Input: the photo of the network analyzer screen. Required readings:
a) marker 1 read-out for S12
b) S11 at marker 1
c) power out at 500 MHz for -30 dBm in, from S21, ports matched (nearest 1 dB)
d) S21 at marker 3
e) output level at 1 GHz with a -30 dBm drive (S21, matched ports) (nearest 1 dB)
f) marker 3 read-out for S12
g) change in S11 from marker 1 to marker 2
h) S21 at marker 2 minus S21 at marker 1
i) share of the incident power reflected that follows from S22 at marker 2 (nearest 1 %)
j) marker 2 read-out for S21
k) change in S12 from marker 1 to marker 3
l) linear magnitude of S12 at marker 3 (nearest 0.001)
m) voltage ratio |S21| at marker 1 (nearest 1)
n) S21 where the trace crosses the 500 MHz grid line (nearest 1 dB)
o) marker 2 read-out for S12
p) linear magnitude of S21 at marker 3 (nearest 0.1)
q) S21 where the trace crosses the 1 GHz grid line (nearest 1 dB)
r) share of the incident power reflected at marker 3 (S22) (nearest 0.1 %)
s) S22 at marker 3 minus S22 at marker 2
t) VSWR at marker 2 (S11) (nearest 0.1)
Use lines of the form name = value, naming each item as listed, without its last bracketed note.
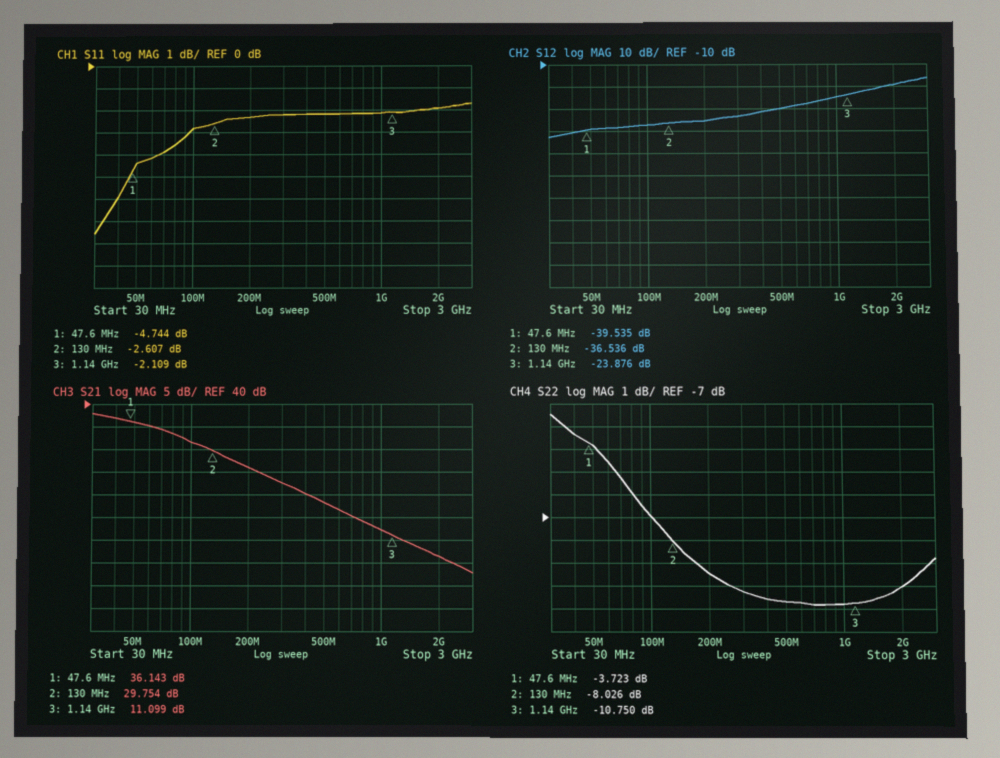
marker 1 read-out for S12 = -39.535 dB
S11 at marker 1 = -4.744 dB
power out at 500 MHz for -30 dBm in, from S21, ports matched = -12 dBm
S21 at marker 3 = 11.099 dB
output level at 1 GHz with a -30 dBm drive (S21, matched ports) = -18 dBm
marker 3 read-out for S12 = -23.876 dB
change in S11 from marker 1 to marker 2 = 2.137 dB
S21 at marker 2 minus S21 at marker 1 = -6.389 dB
share of the incident power reflected that follows from S22 at marker 2 = 16 %
marker 2 read-out for S21 = 29.754 dB
change in S12 from marker 1 to marker 3 = 15.659 dB
linear magnitude of S12 at marker 3 = 0.064
voltage ratio |S21| at marker 1 = 64
S21 where the trace crosses the 500 MHz grid line = 18 dB
marker 2 read-out for S12 = -36.536 dB
linear magnitude of S21 at marker 3 = 3.6
S21 where the trace crosses the 1 GHz grid line = 12 dB
share of the incident power reflected at marker 3 (S22) = 8.4 %
S22 at marker 3 minus S22 at marker 2 = -2.724 dB
VSWR at marker 2 (S11) = 6.7
